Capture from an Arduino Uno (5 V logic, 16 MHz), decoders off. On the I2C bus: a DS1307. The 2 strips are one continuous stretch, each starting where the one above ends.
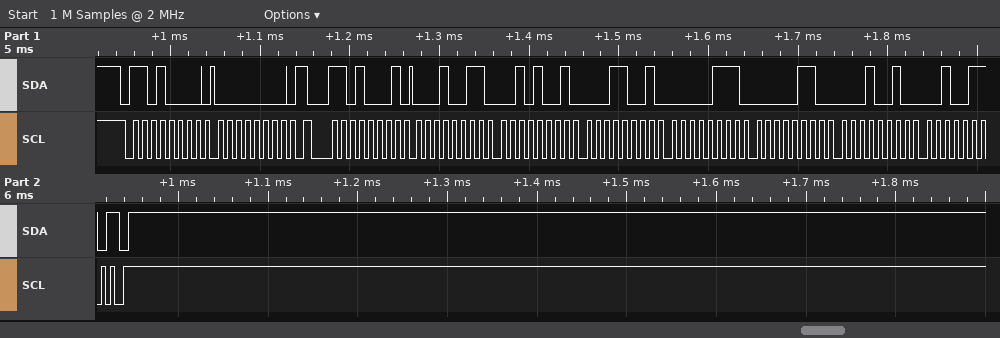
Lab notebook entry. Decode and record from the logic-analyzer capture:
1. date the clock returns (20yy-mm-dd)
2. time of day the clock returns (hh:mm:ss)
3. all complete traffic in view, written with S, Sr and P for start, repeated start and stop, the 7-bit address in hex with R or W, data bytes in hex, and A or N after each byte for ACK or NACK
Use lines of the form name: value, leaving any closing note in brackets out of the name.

date the clock returns: 2026-12-06
time of day the clock returns: 19:29:13
all complete traffic in view, written with S, Sr and P for start, repeated start and stop, the 7-bit address in hex with R or W, data bytes in hex, and A or N after each byte for ACK or NACK: S 68W A 00 A Sr 68R A 13 A 29 A 19 A 07 A 06 A 12 A 26 N P
